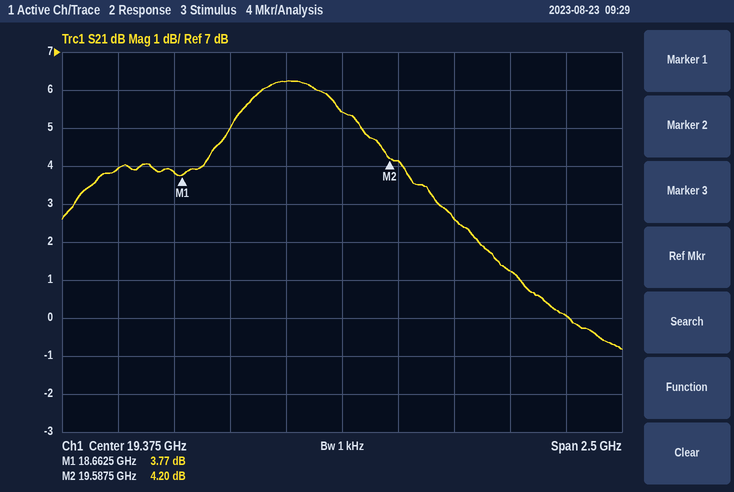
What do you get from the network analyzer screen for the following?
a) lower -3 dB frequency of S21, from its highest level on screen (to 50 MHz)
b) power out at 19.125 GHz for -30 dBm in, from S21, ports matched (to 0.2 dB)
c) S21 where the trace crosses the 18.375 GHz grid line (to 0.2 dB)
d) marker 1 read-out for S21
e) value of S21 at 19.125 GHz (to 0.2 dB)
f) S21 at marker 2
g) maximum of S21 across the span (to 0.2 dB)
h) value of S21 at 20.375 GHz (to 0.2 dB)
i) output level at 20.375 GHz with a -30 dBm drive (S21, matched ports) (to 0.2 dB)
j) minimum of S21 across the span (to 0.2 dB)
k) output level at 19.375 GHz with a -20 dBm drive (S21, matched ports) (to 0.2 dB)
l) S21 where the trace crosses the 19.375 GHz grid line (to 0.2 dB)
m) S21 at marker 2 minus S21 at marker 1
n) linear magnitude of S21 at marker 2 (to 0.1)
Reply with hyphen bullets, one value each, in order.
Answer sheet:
- 18.20 GHz
- -23.8 dBm
- 4.0 dB
- 3.77 dB
- 6.2 dB
- 4.20 dB
- 6.2 dB
- 0.0 dB
- -30.0 dBm
- -0.8 dB
- -14.6 dBm
- 5.4 dB
- 0.43 dB
- 1.6
